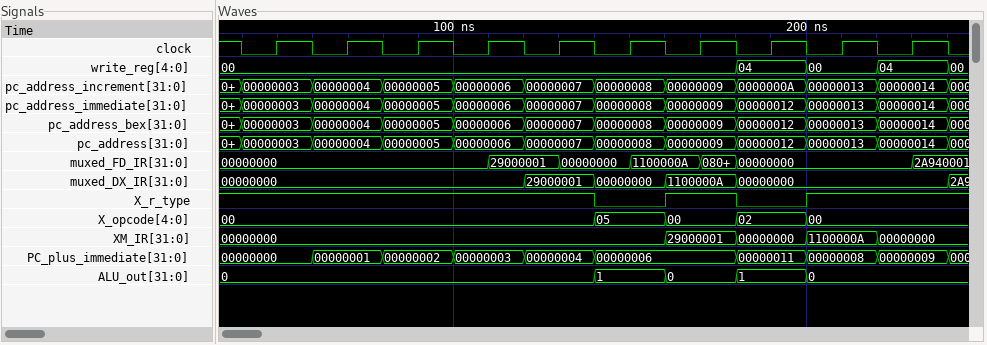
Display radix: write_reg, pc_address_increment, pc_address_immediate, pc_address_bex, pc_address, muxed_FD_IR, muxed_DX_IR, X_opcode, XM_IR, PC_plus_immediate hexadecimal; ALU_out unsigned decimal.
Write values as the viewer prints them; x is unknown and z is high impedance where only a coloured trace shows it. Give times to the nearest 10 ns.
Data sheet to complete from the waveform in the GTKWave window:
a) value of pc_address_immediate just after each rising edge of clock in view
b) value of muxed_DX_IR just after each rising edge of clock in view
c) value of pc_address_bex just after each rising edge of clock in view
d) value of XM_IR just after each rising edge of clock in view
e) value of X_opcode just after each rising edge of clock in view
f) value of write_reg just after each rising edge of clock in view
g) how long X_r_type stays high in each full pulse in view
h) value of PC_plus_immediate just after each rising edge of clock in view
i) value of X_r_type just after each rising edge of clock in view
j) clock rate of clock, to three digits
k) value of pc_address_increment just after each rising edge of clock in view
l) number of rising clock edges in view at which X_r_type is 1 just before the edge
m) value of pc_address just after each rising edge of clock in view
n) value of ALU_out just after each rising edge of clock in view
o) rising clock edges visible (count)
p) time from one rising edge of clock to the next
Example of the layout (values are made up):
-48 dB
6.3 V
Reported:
00000003, 00000004, 00000005, 00000006, 00000007, 00000008, 00000009, 00000012, 00000013, 00000014
00000000, 00000000, 00000000, 00000000, 29000001, 00000000, 1100000A, 00000000, 00000000, 00000000
00000003, 00000004, 00000005, 00000006, 00000007, 00000008, 00000009, 00000012, 00000013, 00000014
00000000, 00000000, 00000000, 00000000, 00000000, 00000000, 29000001, 00000000, 1100000A, 00000000
00, 00, 00, 00, 00, 05, 00, 02, 00, 00
00, 00, 00, 00, 00, 00, 00, 04, 00, 04
20 ns
00000000, 00000001, 00000002, 00000003, 00000004, 00000006, 00000006, 00000011, 00000008, 00000009
1 1 1 1 1 0 1 0 1 1
50.0 MHz
00000003, 00000004, 00000005, 00000006, 00000007, 00000008, 00000009, 0000000A, 00000013, 00000014
8
00000003, 00000004, 00000005, 00000006, 00000007, 00000008, 00000009, 00000012, 00000013, 00000014
0, 0, 0, 0, 0, 1, 0, 1, 0, 0
10
20 ns
